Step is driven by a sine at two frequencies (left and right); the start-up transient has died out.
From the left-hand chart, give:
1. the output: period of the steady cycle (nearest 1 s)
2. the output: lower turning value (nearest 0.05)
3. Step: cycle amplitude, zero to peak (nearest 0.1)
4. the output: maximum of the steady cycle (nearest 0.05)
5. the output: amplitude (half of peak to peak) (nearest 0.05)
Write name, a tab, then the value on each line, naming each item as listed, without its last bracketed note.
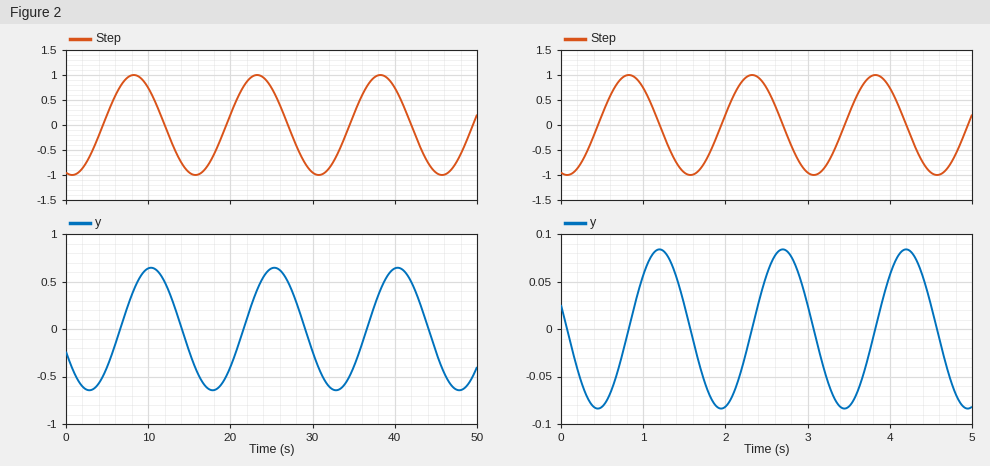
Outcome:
the output: period of the steady cycle	15 s
the output: lower turning value	-0.65
Step: cycle amplitude, zero to peak	1.0
the output: maximum of the steady cycle	0.65
the output: amplitude (half of peak to peak)	0.65
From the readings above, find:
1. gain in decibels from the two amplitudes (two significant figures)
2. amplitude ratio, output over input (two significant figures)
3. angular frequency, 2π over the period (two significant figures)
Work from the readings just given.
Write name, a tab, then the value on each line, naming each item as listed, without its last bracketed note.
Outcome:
gain in decibels from the two amplitudes	-3.7 dB
amplitude ratio, output over input	0.65
angular frequency, 2π over the period	0.42 rad/s
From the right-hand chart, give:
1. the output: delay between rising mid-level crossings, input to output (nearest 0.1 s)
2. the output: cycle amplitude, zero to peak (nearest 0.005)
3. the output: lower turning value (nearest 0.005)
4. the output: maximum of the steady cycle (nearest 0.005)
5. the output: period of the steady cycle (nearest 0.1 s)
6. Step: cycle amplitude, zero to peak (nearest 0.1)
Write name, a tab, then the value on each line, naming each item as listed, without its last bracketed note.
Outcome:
the output: delay between rising mid-level crossings, input to output	0.4 s
the output: cycle amplitude, zero to peak	0.085
the output: lower turning value	-0.085
the output: maximum of the steady cycle	0.085
the output: period of the steady cycle	1.5 s
Step: cycle amplitude, zero to peak	1.0
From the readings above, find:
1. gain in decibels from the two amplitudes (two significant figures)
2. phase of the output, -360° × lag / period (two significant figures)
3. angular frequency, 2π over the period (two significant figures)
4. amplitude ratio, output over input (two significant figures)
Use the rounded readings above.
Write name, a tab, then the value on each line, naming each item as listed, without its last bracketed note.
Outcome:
gain in decibels from the two amplitudes	-21 dB
phase of the output, -360° × lag / period	-96°
angular frequency, 2π over the period	4.2 rad/s
amplitude ratio, output over input	0.085
